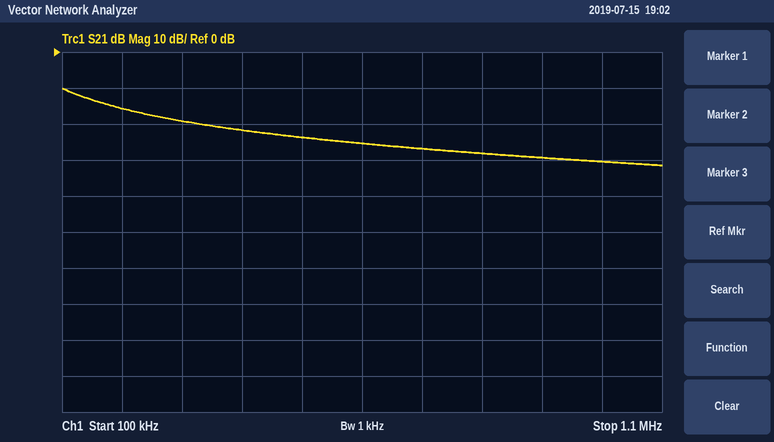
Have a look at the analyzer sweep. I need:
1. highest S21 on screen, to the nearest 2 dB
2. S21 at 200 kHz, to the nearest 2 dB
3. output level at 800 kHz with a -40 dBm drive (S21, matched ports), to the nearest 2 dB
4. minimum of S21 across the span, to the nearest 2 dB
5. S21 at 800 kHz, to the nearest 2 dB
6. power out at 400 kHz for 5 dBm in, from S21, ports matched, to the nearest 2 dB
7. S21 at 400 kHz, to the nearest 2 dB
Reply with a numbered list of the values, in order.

1. -10 dB
2. -16 dB
3. -68 dBm
4. -32 dB
5. -28 dB
6. -16 dBm
7. -22 dB
